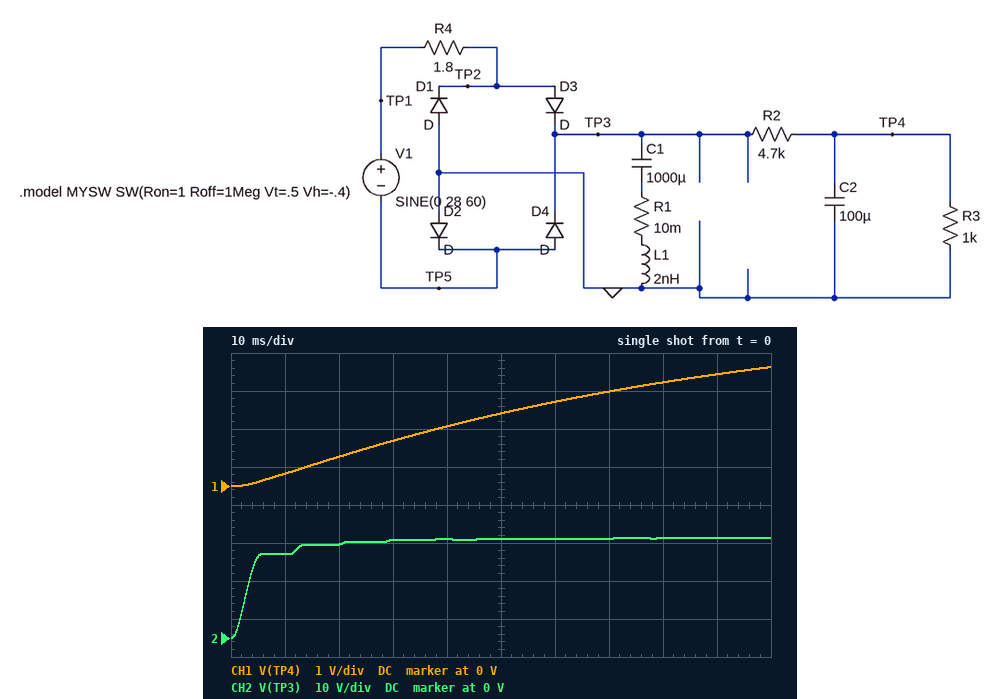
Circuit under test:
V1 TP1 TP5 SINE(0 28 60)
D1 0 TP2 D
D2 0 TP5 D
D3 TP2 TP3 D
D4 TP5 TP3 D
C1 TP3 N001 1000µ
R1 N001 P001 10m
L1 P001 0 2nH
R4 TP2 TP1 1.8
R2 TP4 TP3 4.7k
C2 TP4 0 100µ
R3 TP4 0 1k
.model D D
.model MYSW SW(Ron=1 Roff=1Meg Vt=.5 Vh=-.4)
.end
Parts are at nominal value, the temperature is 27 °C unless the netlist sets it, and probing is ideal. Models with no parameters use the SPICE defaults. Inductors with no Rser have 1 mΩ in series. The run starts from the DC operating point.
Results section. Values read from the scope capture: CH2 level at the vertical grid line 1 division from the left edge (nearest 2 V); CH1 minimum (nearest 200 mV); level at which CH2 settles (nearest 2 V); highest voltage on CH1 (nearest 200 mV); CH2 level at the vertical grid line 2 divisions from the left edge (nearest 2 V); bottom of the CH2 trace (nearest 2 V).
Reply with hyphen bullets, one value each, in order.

- 22 V
- 0 V
- 26 V
- 3.2 V
- 24 V
- 0 V
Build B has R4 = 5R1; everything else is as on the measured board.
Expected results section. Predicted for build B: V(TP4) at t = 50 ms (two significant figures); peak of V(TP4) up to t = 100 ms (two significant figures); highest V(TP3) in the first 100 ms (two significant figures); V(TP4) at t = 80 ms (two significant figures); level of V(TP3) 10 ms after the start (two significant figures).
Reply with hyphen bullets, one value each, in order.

- 1.6 V
- 2.9 V
- 26 V
- 2.5 V
- 15 V
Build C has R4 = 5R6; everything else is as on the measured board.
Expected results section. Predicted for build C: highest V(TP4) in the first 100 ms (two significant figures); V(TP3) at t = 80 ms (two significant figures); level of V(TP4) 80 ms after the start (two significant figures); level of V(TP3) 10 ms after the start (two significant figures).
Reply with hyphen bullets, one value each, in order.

- 2.9 V
- 25 V
- 2.4 V
- 14 V
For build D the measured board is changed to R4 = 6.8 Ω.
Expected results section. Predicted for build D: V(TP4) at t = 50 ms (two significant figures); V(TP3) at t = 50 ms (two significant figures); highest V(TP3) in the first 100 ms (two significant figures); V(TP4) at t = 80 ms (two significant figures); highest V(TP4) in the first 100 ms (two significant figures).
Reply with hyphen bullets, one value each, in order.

- 1.5 V
- 24 V
- 25 V
- 2.4 V
- 2.8 V
